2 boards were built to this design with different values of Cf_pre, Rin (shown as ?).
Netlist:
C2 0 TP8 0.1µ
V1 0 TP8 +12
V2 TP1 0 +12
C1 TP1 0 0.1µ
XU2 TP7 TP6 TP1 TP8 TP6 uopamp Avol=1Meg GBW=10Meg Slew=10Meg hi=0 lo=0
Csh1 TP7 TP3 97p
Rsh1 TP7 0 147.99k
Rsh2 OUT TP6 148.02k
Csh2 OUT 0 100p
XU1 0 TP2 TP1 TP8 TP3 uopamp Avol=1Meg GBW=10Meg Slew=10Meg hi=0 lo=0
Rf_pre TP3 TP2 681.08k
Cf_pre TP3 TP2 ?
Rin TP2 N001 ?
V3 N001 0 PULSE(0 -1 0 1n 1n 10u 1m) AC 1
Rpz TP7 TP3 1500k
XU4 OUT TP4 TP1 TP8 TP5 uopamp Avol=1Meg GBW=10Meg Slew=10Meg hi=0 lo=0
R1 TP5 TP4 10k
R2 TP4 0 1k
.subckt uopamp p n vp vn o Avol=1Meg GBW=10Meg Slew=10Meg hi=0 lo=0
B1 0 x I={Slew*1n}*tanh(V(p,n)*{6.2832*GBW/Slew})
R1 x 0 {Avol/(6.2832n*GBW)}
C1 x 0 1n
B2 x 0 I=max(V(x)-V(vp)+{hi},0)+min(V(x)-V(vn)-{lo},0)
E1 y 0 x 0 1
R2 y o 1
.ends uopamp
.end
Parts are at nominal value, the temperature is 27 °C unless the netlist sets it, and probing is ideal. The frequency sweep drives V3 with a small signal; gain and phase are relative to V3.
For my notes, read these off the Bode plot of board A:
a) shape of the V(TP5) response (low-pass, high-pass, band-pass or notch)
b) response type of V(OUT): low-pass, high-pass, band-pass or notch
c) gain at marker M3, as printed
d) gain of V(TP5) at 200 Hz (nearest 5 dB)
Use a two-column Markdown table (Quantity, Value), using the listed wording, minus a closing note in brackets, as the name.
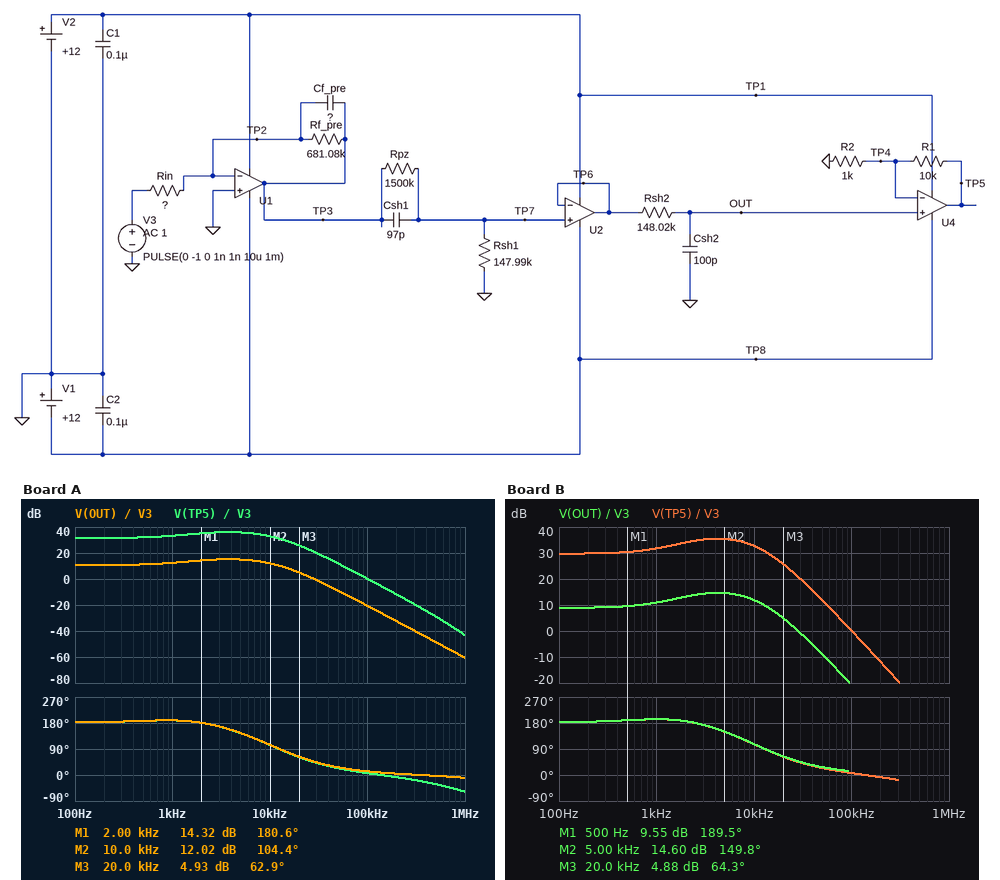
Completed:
| Quantity | Value |
|---|---|
| shape of the V(TP5) response | low-pass |
| response type of V(OUT): low-pass, high-pass, band-pass or notch | low-pass |
| gain at marker M3, as printed | 4.93 dB |
| gain of V(TP5) at 200 Hz | 30 dB |
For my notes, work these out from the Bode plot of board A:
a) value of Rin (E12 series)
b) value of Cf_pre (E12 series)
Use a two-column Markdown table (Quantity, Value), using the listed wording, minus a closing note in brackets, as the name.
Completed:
| Quantity | Value |
|---|---|
| value of Rin | 18 kΩ |
| value of Cf_pre | 100 pF |
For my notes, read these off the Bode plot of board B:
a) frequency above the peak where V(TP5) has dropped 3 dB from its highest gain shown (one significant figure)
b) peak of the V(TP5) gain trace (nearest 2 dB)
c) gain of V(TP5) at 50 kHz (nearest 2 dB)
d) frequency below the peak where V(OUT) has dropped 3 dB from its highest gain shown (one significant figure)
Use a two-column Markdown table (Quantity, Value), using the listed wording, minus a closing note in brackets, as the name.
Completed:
| Quantity | Value |
|---|---|
| frequency above the peak where V(TP5) has dropped 3 dB from its highest gain shown | 10 kHz |
| peak of the V(TP5) gain trace | 36 dB |
| gain of V(TP5) at 50 kHz | 12 dB |
| frequency below the peak where V(OUT) has dropped 3 dB from its highest gain shown | 1 kHz |
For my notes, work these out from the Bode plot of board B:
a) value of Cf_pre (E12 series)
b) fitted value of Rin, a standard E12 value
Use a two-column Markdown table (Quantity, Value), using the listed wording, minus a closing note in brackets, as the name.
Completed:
| Quantity | Value |
|---|---|
| value of Cf_pre | 82 pF |
| fitted value of Rin, a standard E12 value | 22 kΩ |
